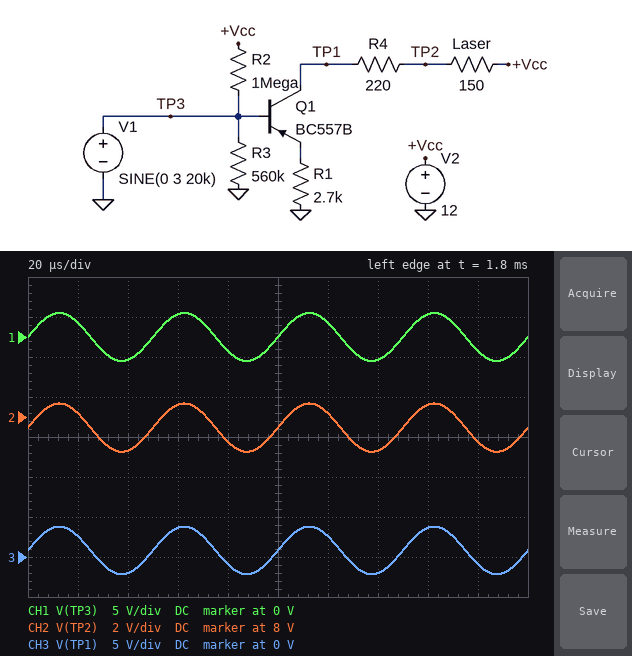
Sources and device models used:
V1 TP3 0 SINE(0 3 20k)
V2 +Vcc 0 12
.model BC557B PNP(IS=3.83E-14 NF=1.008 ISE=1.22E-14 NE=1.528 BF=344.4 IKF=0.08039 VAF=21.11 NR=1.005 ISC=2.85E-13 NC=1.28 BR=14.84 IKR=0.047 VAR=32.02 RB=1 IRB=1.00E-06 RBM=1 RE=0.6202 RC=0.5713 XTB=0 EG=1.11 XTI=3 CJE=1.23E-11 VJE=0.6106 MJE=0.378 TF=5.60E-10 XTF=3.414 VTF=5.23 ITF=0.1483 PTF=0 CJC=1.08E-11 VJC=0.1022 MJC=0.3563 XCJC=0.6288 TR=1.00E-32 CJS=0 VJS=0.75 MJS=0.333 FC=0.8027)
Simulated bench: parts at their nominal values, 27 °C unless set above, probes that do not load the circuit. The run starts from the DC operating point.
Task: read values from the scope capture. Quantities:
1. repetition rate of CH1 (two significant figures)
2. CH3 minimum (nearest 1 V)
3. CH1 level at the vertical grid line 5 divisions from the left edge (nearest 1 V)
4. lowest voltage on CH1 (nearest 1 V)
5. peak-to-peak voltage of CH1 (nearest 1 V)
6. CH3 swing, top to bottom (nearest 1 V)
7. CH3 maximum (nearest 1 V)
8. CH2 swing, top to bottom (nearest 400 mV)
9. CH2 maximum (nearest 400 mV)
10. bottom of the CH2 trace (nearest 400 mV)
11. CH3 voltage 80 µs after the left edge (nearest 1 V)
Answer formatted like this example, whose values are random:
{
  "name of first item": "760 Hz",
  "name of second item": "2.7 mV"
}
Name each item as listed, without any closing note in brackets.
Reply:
{
  "repetition rate of CH1": "20 kHz",
  "CH3 minimum": "-2 V",
  "CH1 level at the vertical grid line 5 divisions from the left edge": "0 V",
  "lowest voltage on CH1": "-3 V",
  "peak-to-peak voltage of CH1": "6 V",
  "CH3 swing, top to bottom": "6 V",
  "CH3 maximum": "4 V",
  "CH2 swing, top to bottom": "2.4 V",
  "CH2 maximum": "8.8 V",
  "bottom of the CH2 trace": "6.4 V",
  "CH3 voltage 80 µs after the left edge": "-1 V"
}
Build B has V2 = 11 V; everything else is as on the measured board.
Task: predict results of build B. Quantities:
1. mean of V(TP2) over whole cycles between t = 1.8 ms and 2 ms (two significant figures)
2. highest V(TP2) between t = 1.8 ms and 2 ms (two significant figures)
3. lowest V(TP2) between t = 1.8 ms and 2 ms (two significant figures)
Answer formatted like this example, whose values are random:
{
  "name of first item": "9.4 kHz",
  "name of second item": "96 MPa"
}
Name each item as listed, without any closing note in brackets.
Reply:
{
  "mean of V(TP2) over whole cycles between t = 1.8 ms and 2 ms": "6.9 V",
  "highest V(TP2) between t = 1.8 ms and 2 ms": "8.1 V",
  "lowest V(TP2) between t = 1.8 ms and 2 ms": "5.7 V"
}
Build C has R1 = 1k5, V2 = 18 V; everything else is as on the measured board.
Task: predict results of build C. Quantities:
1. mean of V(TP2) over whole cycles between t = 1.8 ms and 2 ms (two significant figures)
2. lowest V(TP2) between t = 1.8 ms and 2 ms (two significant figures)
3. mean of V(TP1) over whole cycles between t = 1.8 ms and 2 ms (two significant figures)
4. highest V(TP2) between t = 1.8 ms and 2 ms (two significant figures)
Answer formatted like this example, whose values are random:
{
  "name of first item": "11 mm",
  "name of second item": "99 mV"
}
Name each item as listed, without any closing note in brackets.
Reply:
{
  "mean of V(TP2) over whole cycles between t = 1.8 ms and 2 ms": "11 V",
  "lowest V(TP2) between t = 1.8 ms and 2 ms": "9.8 V",
  "mean of V(TP1) over whole cycles between t = 1.8 ms and 2 ms": "860 mV",
  "highest V(TP2) between t = 1.8 ms and 2 ms": "12 V"
}
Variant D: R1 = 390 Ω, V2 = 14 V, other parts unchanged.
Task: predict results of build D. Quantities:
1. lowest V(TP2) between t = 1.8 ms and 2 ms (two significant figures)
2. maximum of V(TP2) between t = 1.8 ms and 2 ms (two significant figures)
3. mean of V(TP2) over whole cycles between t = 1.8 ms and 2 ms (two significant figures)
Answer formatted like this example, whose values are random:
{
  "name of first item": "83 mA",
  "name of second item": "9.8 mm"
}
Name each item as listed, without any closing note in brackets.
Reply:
{
  "lowest V(TP2) between t = 1.8 ms and 2 ms": "7.5 V",
  "maximum of V(TP2) between t = 1.8 ms and 2 ms": "9.9 V",
  "mean of V(TP2) over whole cycles between t = 1.8 ms and 2 ms": "8.7 V"
}
